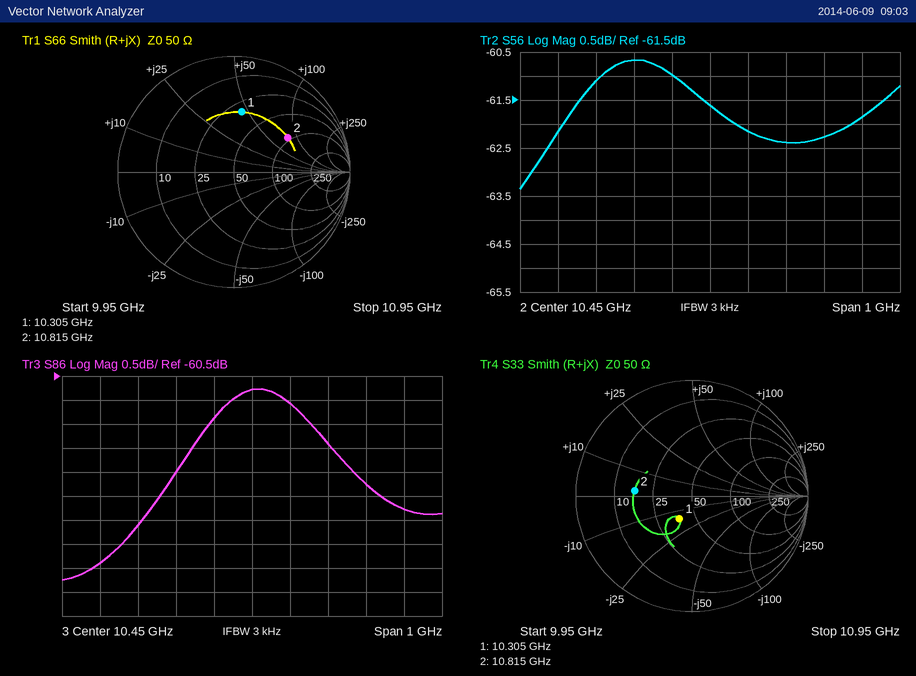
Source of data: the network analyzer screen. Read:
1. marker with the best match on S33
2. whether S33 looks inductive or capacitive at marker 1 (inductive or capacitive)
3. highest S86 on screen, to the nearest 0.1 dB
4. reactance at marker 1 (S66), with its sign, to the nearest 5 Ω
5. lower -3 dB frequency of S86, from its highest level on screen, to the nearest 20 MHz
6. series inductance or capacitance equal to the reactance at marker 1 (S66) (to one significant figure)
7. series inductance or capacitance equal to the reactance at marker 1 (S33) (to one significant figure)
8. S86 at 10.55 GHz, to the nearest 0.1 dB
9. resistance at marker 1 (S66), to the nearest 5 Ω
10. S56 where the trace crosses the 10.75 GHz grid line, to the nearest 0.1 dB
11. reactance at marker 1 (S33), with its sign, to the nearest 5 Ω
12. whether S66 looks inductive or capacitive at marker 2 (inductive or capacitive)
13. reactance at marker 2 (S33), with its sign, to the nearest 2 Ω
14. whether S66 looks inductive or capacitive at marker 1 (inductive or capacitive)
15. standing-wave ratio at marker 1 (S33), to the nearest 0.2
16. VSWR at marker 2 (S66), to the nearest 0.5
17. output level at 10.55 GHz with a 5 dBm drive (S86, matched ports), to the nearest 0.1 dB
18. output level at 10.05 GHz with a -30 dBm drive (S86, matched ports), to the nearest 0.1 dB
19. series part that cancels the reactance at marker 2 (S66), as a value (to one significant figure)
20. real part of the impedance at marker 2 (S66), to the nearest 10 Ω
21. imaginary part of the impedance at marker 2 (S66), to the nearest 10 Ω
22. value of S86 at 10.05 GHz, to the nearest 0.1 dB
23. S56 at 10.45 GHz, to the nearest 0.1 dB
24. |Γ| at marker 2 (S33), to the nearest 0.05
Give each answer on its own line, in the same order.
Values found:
marker 1
capacitive
-60.8 dB
+45 Ω
10.14 GHz
700 pH
1 pF
-61.1 dB
30 Ω
-62.3 dB
-15 Ω
inductive
+2 Ω
inductive
1.6
3.5
-56.1 dBm
-94.4 dBm
200 fF
90 Ω
+80 Ω
-64.4 dB
-61.6 dB
0.50
